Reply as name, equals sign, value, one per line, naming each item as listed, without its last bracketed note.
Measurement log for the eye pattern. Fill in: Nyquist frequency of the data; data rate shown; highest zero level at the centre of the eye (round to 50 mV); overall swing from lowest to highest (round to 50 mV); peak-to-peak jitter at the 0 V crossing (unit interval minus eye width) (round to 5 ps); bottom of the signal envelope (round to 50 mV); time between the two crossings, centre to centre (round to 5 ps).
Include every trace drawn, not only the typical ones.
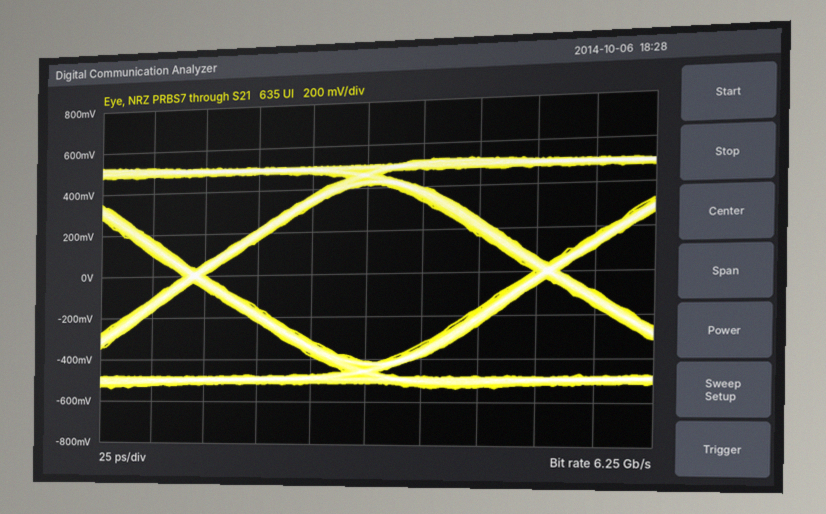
Nyquist frequency of the data = 3.125 GHz
data rate shown = 6.25 Gb/s
highest zero level at the centre of the eye = -400 mV
overall swing from lowest to highest = 1.05 V
peak-to-peak jitter at the 0 V crossing (unit interval minus eye width) = 10 ps
bottom of the signal envelope = -550 mV
time between the two crossings, centre to centre = 160 ps
